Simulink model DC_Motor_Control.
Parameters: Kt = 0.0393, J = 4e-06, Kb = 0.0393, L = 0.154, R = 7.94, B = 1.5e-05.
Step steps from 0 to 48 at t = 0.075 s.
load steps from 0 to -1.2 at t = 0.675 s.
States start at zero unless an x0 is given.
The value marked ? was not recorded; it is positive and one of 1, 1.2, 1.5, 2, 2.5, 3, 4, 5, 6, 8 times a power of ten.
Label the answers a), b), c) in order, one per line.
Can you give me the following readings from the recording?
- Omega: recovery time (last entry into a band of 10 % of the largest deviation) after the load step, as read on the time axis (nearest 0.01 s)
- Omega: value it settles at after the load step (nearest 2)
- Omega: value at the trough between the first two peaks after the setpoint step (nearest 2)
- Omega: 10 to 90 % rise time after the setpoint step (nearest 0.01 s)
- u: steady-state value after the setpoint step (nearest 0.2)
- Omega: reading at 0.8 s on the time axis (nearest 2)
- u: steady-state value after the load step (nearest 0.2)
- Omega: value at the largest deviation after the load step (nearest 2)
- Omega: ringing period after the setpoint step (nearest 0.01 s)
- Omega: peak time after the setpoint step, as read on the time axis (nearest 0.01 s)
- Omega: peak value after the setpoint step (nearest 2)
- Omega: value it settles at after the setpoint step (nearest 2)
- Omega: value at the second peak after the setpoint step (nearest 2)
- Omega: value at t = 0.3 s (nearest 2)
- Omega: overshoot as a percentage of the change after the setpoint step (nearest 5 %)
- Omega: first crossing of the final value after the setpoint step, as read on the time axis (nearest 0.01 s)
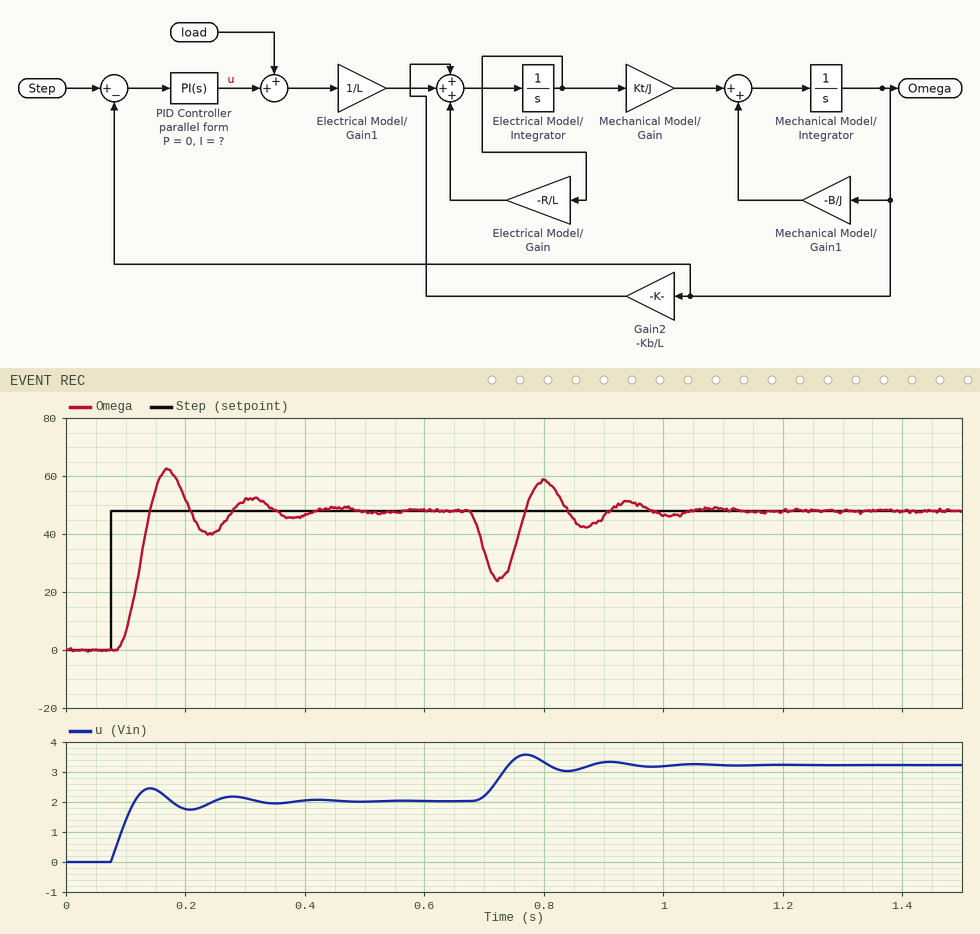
a) 0.96 s
b) 48
c) 40
d) 0.04 s
e) 2.0
f) 58
g) 3.2
h) 24
i) 0.14 s
j) 0.17 s
k) 62
l) 48
m) 52
n) 52
o) 30 %
p) 0.14 s
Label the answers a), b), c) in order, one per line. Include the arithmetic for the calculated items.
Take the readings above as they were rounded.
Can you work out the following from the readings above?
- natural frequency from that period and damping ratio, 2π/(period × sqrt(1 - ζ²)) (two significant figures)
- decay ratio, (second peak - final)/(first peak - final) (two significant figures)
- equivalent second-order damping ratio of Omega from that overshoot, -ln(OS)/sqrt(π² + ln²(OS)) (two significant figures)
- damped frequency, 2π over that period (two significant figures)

a) 2π / (0.14 × sqrt(1 - 0.36²)) = 48 rad/s
b) (52 - 48) / (62 - 48) = 0.29
c) ln(0.3) = -1.204; 1.204 / sqrt(9.870 + 1.450) = 0.36
d) 2π / 0.14 = 45 rad/s
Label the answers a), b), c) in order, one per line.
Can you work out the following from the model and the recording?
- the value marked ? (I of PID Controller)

a) 1.2
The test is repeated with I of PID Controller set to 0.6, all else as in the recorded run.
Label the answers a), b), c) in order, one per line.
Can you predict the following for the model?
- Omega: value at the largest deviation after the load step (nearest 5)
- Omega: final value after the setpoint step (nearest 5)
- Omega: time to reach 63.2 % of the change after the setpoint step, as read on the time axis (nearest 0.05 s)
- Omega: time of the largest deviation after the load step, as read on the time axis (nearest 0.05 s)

a) 20
b) 50
c) 0.15 s
d) 0.75 s
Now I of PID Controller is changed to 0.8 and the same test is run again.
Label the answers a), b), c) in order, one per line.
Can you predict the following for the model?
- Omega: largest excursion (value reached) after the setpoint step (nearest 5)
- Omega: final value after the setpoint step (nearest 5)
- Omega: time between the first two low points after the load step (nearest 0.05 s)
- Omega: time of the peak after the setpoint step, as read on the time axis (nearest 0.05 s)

a) 50
b) 50
c) 0.15 s
d) 0.20 s
